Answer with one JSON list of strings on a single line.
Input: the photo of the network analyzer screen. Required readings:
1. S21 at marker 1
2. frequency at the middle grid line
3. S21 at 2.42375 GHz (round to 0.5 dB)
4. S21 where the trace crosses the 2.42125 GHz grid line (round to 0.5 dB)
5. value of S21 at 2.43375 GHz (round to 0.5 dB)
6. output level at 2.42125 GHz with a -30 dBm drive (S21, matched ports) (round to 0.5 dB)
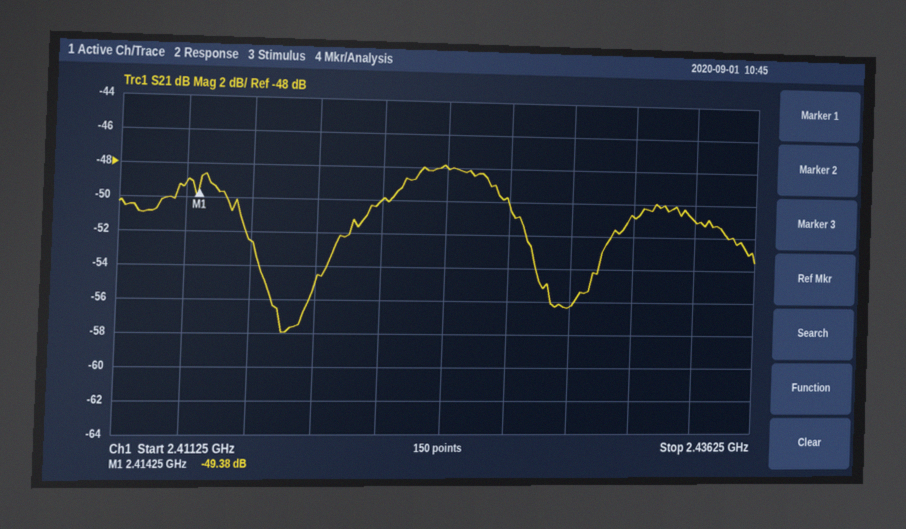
["-49.38 dB", "2.42375 GHz", "-48.0 dB", "-50.0 dB", "-51.0 dB", "-80.0 dBm"]
